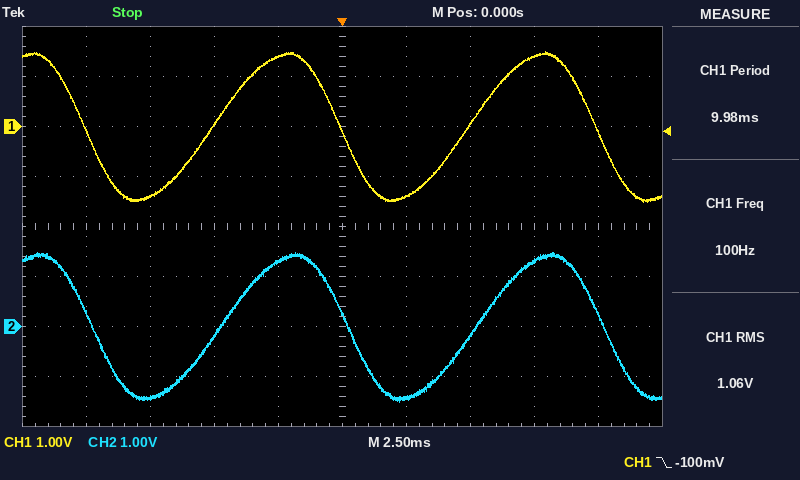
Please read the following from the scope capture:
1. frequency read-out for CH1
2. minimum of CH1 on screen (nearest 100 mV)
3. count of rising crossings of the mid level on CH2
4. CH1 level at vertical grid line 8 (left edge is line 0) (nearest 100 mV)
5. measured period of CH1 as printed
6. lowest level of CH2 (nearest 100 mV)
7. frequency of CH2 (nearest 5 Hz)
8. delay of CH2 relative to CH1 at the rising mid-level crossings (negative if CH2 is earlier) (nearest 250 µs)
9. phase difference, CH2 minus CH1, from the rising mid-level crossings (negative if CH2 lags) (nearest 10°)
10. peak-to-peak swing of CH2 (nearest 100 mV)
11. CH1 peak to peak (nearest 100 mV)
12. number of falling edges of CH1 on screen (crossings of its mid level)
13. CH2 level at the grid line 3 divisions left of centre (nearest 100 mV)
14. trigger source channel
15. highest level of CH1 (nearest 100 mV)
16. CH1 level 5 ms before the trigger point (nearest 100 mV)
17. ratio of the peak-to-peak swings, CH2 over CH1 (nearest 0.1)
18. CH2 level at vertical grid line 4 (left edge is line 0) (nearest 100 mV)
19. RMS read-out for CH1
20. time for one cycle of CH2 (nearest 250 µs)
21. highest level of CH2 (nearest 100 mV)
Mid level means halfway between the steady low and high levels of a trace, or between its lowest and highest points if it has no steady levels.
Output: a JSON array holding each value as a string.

["100 Hz", "-1.5 V", "2", "1.4 V", "9.98 ms", "-1.5 V", "100 Hz", "+250 µs", "-10°", "3.0 V", "3.0 V", "3", "-1.4 V", "CH1", "1.5 V", "0.0 V", "1.0", "1.3 V", "1.06 V", "10.00 ms", "1.5 V"]
